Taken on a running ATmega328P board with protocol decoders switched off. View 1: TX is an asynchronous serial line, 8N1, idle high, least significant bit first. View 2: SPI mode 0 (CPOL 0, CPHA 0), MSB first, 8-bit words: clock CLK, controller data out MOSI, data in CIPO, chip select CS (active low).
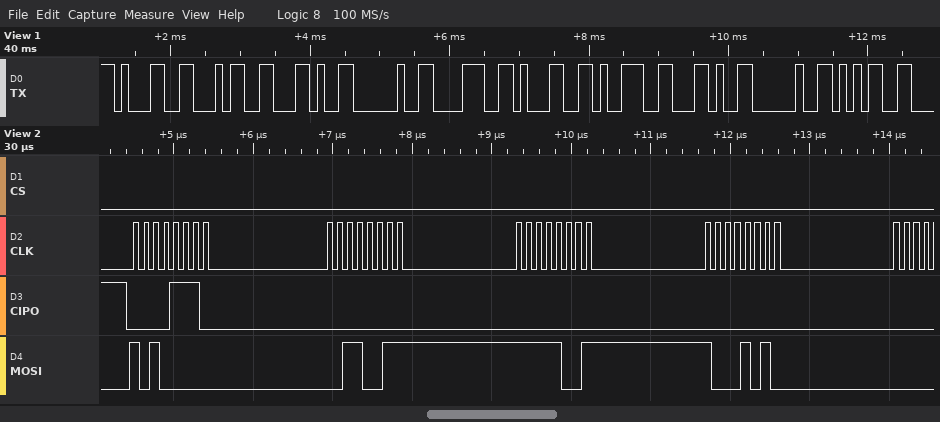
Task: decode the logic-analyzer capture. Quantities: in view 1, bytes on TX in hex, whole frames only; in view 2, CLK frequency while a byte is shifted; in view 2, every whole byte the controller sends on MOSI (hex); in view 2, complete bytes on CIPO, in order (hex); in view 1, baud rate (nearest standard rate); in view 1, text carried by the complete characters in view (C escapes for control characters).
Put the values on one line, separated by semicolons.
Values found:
31 34 2C 20 38 31 39 2C 20 35; 8 MHz; A0 33 F9 8A; 0E 00 00 00; 9600 baud; "14, 819, 5"
